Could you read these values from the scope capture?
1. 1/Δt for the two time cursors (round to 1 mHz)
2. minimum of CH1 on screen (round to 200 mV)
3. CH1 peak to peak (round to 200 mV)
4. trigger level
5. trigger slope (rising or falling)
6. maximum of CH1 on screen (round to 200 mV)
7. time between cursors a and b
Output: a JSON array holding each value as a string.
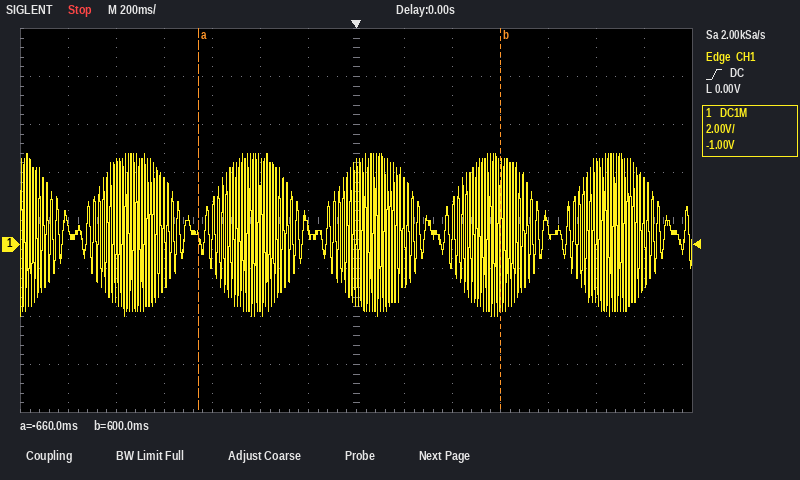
["794 mHz", "-3.0 V", "6.8 V", "0.00 V", "rising", "3.8 V", "1.26 s"]
